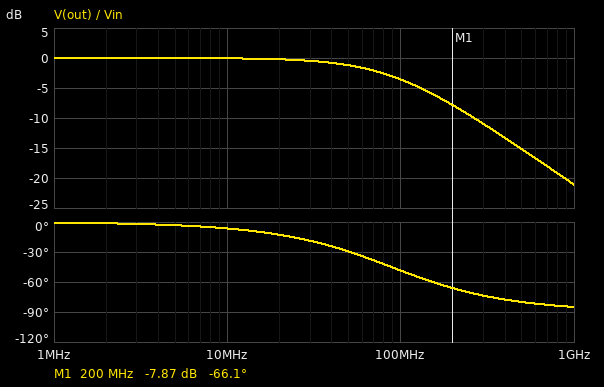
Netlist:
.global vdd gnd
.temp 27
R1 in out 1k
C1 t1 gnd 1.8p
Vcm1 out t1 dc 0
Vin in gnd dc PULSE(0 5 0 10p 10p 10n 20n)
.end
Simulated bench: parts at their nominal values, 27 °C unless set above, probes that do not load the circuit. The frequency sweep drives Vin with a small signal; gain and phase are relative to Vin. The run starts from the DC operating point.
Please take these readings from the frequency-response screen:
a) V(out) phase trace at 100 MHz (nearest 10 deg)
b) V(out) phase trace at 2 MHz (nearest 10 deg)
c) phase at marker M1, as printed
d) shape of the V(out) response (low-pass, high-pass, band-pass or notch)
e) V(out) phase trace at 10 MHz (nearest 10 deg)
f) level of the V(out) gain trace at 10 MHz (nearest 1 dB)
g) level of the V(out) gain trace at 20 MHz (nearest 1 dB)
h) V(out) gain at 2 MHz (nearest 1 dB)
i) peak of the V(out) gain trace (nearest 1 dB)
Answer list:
-50 deg
0 deg
-66.1 deg
low-pass
-10 deg
0 dB
0 dB
0 dB
0 dB
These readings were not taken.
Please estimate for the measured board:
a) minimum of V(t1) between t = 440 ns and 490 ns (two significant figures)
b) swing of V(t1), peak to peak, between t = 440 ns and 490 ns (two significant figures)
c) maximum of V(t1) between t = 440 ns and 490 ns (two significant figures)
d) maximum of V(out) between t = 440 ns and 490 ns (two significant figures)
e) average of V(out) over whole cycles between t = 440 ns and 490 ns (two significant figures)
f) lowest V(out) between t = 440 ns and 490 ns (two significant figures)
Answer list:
19 mV
5.0 V
5.0 V
5.0 V
2.5 V
19 mV
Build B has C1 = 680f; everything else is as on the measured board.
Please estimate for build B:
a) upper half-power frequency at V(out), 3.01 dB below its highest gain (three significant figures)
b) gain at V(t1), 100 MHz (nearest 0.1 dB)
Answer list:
234 MHz
-0.7 dB
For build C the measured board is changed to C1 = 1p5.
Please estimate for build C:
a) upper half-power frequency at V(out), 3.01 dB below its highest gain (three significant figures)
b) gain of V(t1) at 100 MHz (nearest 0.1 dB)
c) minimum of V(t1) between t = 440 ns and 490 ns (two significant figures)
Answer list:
106 MHz
-2.8 dB
6.4 mV
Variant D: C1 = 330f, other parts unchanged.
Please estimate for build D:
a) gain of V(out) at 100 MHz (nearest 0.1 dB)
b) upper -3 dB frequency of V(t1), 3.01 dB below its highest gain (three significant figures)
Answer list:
-0.2 dB
482 MHz
